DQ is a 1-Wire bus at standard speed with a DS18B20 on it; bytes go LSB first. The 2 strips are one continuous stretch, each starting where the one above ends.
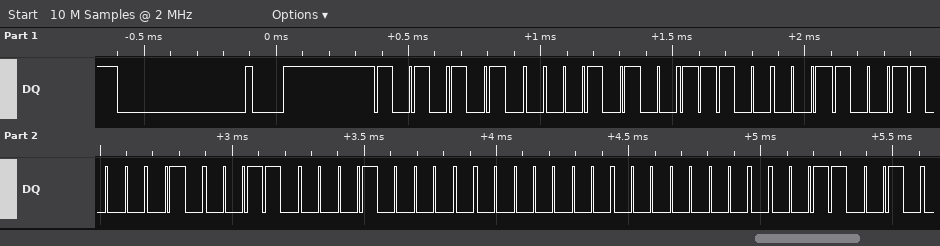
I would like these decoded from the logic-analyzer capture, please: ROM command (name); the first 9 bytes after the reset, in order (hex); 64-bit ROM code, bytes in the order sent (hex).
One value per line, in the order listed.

Match ROM
55 28 87 19 62 08 00 00 4C
28 87 19 62 08 00 00 4C
